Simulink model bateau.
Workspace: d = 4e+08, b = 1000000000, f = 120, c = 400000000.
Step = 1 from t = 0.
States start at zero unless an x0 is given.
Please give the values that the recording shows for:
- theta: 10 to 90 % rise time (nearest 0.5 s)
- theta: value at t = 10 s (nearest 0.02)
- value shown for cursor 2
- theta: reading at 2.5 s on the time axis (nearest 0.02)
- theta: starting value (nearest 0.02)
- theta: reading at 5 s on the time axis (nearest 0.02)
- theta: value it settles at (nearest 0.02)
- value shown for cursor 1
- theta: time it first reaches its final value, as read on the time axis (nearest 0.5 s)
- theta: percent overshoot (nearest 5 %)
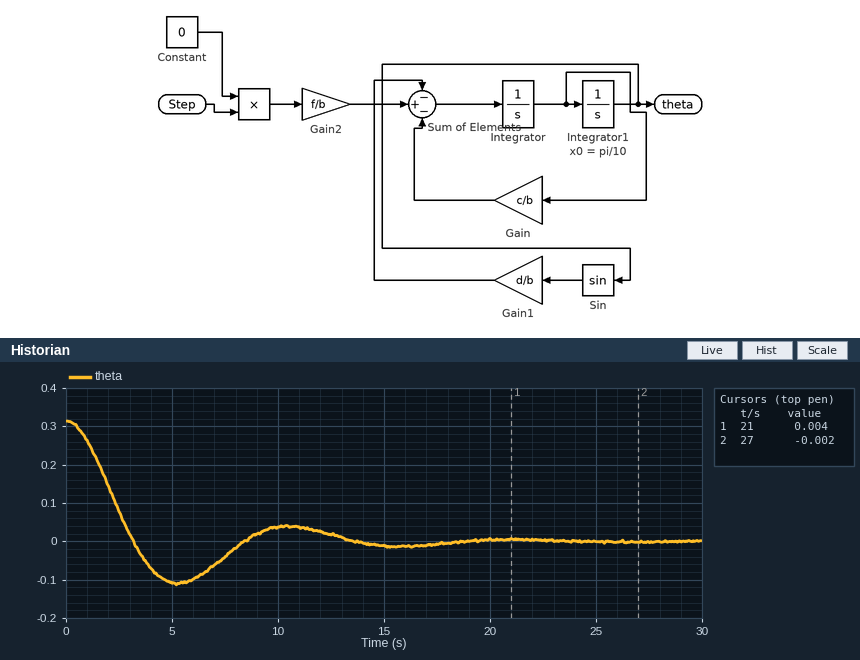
2.0 s
0.04
-0.002
0.08
0.32
-0.10
0.00
0.004
3.0 s
35 %
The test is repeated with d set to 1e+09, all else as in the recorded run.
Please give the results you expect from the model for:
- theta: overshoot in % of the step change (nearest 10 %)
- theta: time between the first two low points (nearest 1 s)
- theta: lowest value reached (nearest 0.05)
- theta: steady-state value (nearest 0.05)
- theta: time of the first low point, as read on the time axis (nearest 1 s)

50 %
6 s
-0.15
0.00
3 s
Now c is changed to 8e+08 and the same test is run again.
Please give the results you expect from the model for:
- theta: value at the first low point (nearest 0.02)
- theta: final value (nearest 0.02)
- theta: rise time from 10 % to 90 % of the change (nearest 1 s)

-0.02
0.00
3 s
